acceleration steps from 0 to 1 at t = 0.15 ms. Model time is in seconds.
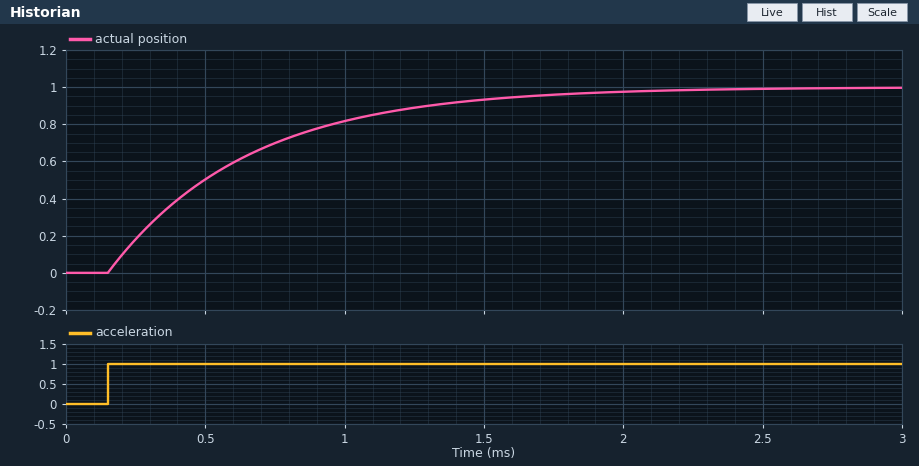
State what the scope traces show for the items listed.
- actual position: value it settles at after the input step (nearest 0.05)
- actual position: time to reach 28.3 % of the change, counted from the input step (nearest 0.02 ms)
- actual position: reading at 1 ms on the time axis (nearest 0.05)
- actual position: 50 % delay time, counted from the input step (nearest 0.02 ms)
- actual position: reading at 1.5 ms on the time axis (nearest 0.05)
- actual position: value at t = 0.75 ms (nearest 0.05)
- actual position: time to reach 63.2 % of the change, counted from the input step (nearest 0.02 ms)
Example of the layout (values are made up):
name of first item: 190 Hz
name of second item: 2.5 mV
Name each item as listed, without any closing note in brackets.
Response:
actual position: value it settles at after the input step: 1.00
actual position: time to reach 28.3 % of the change, counted from the input step: 0.16 ms
actual position: reading at 1 ms on the time axis: 0.80
actual position: 50 % delay time, counted from the input step: 0.34 ms
actual position: reading at 1.5 ms on the time axis: 0.95
actual position: value at t = 0.75 ms: 0.70
actual position: time to reach 63.2 % of the change, counted from the input step: 0.50 ms
